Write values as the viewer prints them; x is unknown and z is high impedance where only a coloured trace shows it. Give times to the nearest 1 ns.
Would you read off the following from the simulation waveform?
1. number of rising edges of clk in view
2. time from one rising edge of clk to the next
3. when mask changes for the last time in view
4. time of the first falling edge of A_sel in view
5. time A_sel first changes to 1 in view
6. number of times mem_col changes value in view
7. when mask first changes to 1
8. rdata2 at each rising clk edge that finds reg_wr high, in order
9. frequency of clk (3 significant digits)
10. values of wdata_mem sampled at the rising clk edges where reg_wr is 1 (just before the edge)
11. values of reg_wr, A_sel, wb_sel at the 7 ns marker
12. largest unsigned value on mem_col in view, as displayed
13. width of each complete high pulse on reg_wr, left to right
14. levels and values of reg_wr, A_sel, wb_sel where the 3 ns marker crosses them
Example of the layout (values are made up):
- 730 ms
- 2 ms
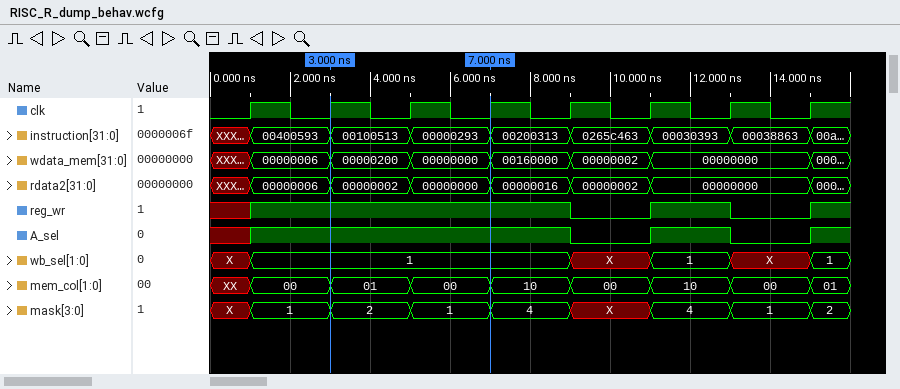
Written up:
- 8
- 2 ns
- 15 ns
- 9 ns
- 1 ns
- 8
- 1 ns
- 00000006, 00000002, 00000000, 00000016, 00000000
- 500 MHz
- 00000006, 00000200, 00000000, 00160000, 00000000
- reg_wr=1, A_sel=1, wb_sel=1
- 10
- 2 ns
- reg_wr=1, A_sel=1, wb_sel=1
